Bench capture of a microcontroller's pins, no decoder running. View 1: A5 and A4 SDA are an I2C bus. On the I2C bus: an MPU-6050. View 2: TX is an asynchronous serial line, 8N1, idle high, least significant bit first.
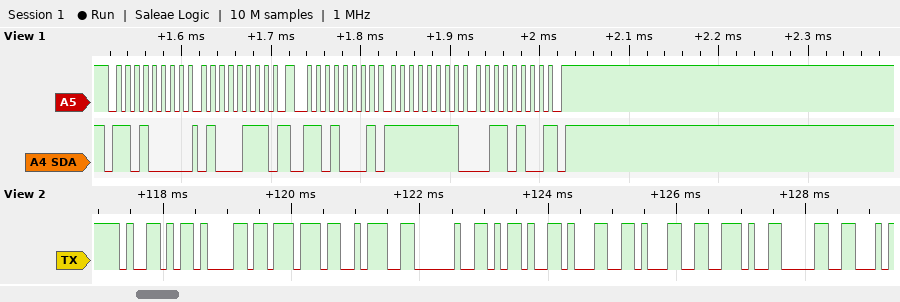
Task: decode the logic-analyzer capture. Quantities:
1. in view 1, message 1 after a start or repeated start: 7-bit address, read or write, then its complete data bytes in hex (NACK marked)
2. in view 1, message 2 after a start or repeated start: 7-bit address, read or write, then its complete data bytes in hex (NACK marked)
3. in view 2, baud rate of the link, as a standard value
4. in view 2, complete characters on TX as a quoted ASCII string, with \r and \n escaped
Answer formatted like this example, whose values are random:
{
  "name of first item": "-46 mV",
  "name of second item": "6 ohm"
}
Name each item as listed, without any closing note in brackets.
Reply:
{
  "in view 1, message 1 after a start or repeated start: 7-bit address, read or write, then its complete data bytes in hex": "0x68 write: 47",
  "in view 1, message 2 after a start or repeated start: 7-bit address, read or write, then its complete data bytes in hex": "0x68 read: FF 34 NACK",
  "in view 2, baud rate of the link, as a standard value": "9600 baud",
  "in view 2, complete characters on TX as a quoted ASCII string, with \\r and \\n escaped": "\"Yaw: -11.0\""
}
